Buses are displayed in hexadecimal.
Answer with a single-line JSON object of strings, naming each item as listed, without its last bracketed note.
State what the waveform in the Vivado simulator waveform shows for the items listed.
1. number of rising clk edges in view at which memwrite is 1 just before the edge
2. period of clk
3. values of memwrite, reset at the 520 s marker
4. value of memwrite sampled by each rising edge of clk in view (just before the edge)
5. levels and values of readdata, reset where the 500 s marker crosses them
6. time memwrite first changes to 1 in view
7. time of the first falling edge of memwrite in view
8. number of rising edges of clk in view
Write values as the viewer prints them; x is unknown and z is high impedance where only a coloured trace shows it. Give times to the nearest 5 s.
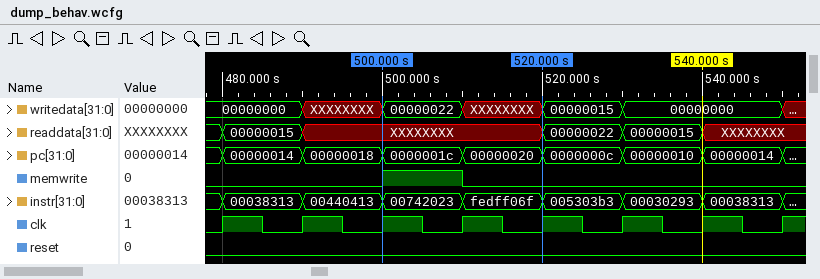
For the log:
{"number of rising clk edges in view at which memwrite is 1 just before the edge": "1", "period of clk": "10 s", "values of memwrite, reset at the 520 s marker": "memwrite=0, reset=0", "value of memwrite sampled by each rising edge of clk in view": "0 0 0 1 0 0 0 0", "levels and values of readdata, reset where the 500 s marker crosses them": "readdata=XXXXXXXX, reset=0", "time memwrite first changes to 1 in view": "500 s", "time of the first falling edge of memwrite in view": "510 s", "number of rising edges of clk in view": "8"}
